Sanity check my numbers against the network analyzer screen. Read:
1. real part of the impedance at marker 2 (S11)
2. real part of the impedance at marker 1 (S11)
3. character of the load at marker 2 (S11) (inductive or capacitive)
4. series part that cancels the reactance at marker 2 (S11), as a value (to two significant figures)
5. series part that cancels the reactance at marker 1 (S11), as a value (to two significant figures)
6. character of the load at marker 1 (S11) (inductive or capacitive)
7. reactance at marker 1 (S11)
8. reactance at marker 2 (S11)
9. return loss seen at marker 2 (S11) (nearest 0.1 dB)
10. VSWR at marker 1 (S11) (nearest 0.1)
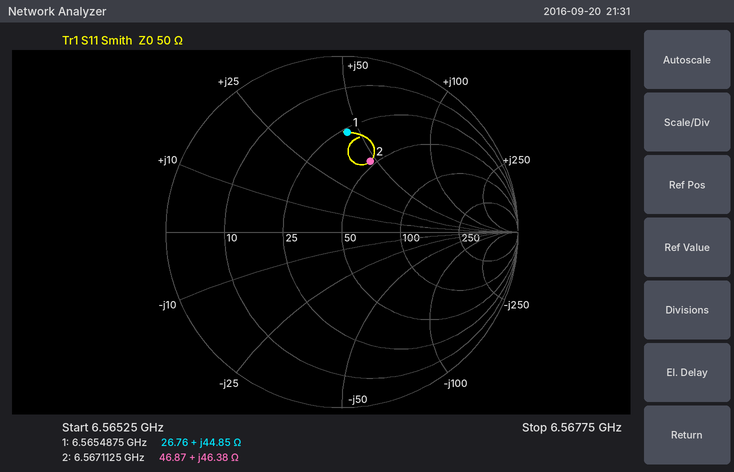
46.87 Ω
26.76 Ω
inductive
520 fF
540 fF
inductive
+44.85 Ω
+46.38 Ω
7.3 dB
3.6
